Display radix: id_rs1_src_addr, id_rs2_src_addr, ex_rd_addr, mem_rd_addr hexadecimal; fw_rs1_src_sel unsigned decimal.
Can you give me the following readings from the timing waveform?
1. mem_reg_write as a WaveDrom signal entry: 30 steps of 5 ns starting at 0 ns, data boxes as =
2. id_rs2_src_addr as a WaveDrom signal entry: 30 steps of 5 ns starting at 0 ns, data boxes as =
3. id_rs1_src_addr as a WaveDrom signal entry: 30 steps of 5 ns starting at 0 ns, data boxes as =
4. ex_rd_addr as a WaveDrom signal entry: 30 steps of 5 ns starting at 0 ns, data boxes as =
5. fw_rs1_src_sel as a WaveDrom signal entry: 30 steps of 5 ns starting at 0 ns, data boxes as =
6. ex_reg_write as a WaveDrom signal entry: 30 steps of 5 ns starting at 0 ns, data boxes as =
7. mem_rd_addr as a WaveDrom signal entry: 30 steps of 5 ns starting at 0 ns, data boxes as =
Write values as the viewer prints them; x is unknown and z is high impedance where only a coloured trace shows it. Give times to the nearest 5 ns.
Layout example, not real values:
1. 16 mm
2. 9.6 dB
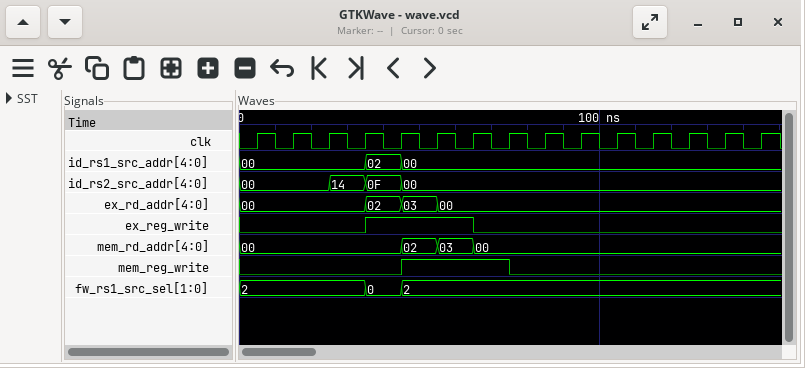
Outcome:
1. {name: 'mem_reg_write', wave: '0........1.....0..............'}
2. {name: 'id_rs2_src_addr', wave: '=....=.=.=....................', data: '00 14 0F 00'}
3. {name: 'id_rs1_src_addr', wave: '=......=.=....................', data: '00 02 00'}
4. {name: 'ex_rd_addr', wave: '=......=.=.=..................', data: '00 02 03 00'}
5. {name: 'fw_rs1_src_sel', wave: '=......=.=....................', data: '2 0 2'}
6. {name: 'ex_reg_write', wave: '0......1.....0................'}
7. {name: 'mem_rd_addr', wave: '=........=.=.=................', data: '00 02 03 00'}
